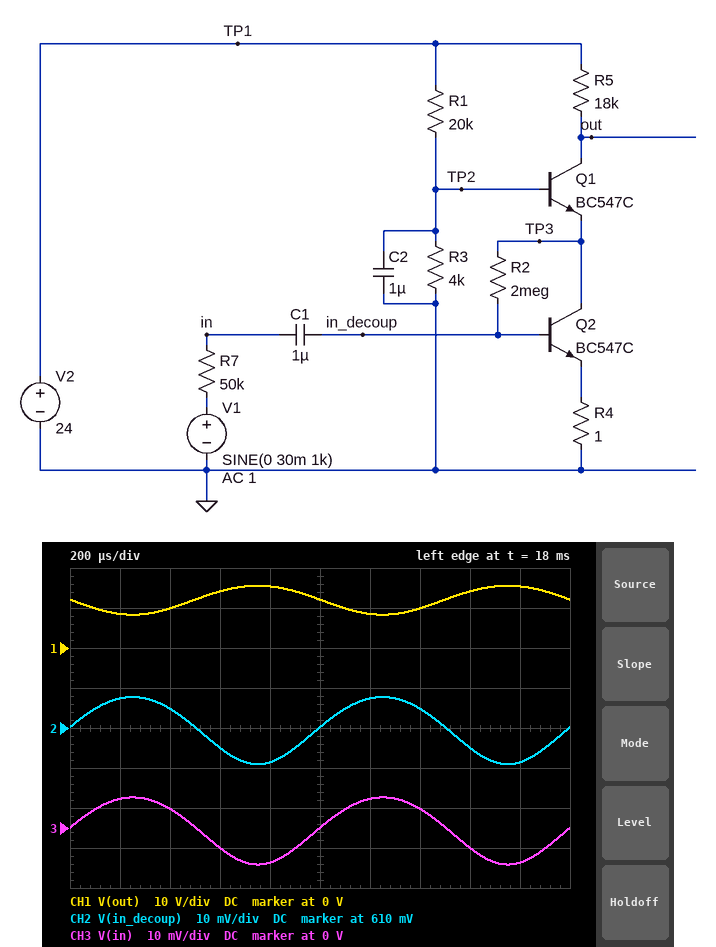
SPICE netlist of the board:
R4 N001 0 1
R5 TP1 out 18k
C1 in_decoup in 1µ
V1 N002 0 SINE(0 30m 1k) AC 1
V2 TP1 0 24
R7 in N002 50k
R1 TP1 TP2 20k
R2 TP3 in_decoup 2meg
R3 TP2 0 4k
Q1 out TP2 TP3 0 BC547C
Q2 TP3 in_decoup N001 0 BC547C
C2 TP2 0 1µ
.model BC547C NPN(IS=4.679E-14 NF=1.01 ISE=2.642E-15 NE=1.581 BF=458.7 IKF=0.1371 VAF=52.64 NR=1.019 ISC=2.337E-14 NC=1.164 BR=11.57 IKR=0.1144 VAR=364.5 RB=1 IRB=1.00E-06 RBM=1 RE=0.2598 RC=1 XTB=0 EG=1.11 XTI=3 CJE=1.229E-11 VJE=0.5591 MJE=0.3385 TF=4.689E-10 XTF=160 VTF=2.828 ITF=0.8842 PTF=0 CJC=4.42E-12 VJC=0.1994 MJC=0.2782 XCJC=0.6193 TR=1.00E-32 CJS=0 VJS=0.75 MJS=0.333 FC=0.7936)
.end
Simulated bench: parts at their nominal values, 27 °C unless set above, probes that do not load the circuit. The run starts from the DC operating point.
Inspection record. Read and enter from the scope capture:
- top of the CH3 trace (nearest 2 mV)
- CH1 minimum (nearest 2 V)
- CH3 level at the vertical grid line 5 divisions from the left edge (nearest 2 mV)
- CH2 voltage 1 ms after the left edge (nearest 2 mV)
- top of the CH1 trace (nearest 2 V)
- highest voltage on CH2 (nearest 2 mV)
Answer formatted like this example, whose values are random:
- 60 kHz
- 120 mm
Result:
- 8 mV
- 8 V
- 0 V
- 610 mV
- 16 V
- 618 mV
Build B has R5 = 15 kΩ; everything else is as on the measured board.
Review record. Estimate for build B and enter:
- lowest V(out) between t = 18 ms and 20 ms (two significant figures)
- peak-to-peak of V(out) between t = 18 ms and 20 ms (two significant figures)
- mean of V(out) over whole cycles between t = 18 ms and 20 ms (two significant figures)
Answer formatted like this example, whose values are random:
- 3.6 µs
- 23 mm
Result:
- 11 V
- 6.0 V
- 14 V
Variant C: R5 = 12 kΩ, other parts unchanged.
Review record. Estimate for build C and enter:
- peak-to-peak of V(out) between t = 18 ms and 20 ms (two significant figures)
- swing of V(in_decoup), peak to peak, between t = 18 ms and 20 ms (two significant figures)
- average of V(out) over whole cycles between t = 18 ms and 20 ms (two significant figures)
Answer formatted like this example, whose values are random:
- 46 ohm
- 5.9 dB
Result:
- 4.8 V
- 17 mV
- 16 V
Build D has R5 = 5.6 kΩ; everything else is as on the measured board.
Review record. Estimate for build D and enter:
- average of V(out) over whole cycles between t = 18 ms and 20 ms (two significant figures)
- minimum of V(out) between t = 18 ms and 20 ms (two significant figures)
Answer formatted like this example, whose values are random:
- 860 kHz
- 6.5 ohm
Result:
- 20 V
- 19 V
